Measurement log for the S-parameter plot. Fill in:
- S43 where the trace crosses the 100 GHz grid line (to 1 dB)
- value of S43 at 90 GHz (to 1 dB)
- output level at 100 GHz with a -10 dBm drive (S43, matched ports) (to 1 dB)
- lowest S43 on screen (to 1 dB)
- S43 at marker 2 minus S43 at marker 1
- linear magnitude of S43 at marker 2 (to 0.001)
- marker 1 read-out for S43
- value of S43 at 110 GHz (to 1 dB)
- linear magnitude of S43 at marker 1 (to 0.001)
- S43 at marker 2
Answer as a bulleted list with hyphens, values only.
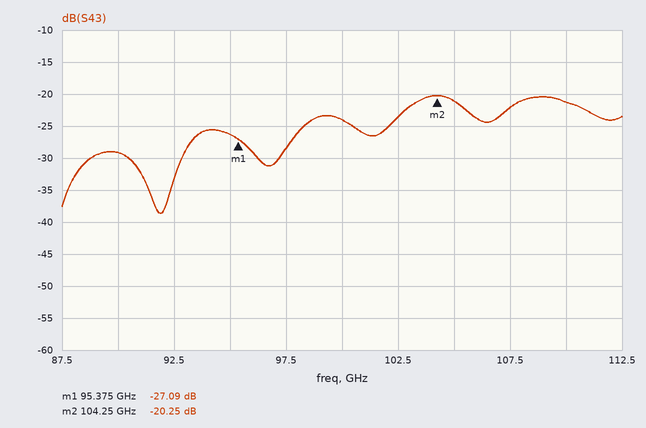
- -24 dB
- -29 dB
- -34 dBm
- -39 dB
- 6.84 dB
- 0.097
- -27.09 dB
- -21 dB
- 0.044
- -20.25 dB
